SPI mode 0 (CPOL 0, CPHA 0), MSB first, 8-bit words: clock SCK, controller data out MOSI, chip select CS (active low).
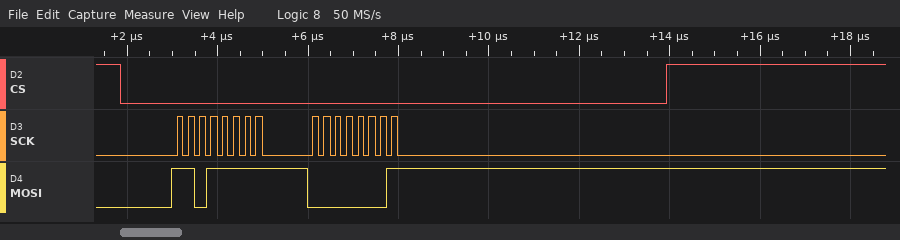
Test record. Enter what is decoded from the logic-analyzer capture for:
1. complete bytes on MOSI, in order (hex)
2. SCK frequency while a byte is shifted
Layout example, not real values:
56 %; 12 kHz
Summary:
DF 01; 4 MHz
